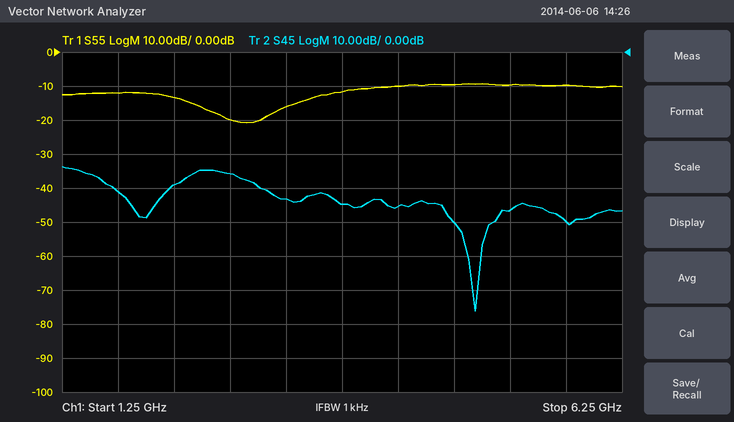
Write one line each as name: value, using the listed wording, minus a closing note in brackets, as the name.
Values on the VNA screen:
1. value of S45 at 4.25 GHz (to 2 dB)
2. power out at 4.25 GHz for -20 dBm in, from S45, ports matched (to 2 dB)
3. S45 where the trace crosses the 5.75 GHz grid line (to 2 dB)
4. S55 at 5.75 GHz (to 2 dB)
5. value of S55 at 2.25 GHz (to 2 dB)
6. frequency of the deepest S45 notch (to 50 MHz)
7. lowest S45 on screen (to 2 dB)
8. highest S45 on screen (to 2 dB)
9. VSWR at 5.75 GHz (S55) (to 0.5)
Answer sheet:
value of S45 at 4.25 GHz: -46 dB
power out at 4.25 GHz for -20 dBm in, from S45, ports matched: -66 dBm
S45 where the trace crosses the 5.75 GHz grid line: -50 dB
S55 at 5.75 GHz: -10 dB
value of S55 at 2.25 GHz: -14 dB
frequency of the deepest S45 notch: 4.95 GHz
lowest S45 on screen: -76 dB
highest S45 on screen: -34 dB
VSWR at 5.75 GHz (S55): 2.0
